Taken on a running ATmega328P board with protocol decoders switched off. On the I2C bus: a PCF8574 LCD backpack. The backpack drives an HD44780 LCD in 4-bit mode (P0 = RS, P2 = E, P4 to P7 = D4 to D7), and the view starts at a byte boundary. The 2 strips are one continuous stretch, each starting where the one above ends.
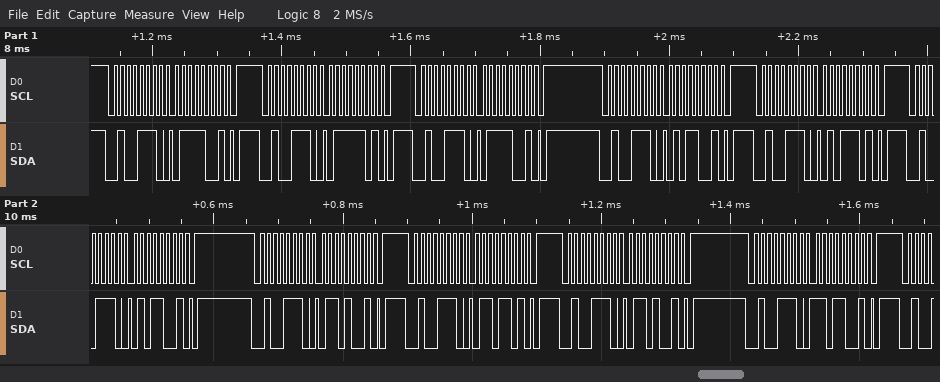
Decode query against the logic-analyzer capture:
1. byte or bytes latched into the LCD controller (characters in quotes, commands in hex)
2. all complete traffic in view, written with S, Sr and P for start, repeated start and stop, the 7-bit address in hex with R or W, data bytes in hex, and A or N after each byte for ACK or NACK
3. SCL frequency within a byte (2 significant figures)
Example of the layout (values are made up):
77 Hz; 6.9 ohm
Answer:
'u'; S 27W A 79 A P S 27W A 7D A P S 27W A 79 A P S 27W A 59 A P S 27W A 5D A P S 27W A 59 A P S 27W A 69 A P S 27W A 6D A P S 27W A 69 A P S 27W A D9 A P; 100 kHz
